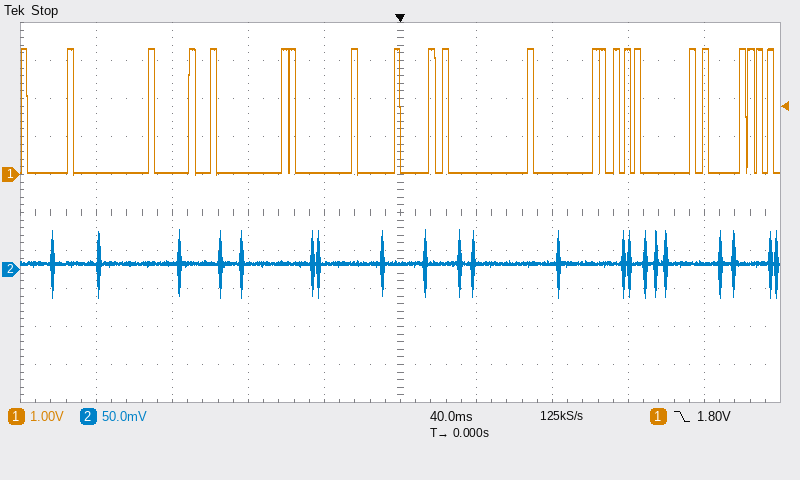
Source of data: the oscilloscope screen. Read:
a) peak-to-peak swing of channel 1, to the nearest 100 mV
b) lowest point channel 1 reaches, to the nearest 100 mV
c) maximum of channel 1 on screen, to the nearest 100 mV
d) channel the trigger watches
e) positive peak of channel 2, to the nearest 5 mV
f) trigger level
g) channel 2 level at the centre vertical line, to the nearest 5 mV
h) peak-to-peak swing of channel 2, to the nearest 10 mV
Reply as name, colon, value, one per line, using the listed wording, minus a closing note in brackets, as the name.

peak-to-peak swing of channel 1, to the nearest 100 mV: 3.3 V
lowest point channel 1 reaches, to the nearest 100 mV: 0.0 V
maximum of channel 1 on screen, to the nearest 100 mV: 3.3 V
channel the trigger watches: channel 1
positive peak of channel 2, to the nearest 5 mV: 55 mV
trigger level: 1.80 V
channel 2 level at the centre vertical line, to the nearest 5 mV: 10 mV
peak-to-peak swing of channel 2, to the nearest 10 mV: 90 mV
